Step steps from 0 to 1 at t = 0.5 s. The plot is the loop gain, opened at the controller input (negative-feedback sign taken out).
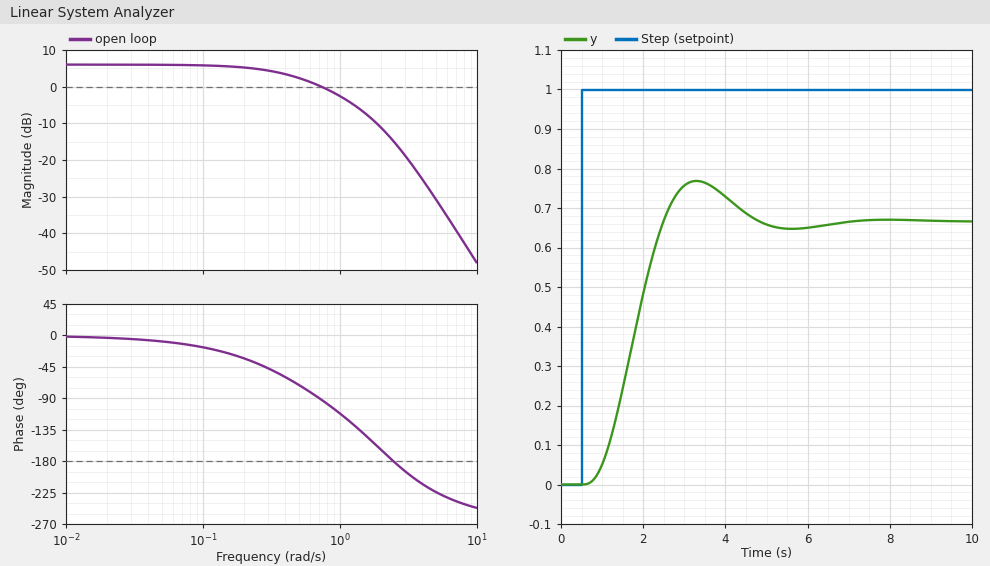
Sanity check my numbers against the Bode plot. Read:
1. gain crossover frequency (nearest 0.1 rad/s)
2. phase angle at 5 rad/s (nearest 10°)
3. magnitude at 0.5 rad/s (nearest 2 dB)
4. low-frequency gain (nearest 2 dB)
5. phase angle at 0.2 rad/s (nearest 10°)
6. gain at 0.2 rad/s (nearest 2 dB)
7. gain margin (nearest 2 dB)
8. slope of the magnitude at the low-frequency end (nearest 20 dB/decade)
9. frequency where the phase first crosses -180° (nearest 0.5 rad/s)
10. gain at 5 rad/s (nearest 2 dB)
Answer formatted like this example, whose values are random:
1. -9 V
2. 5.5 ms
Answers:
1. 0.7 rad/s
2. -220°
3. 2 dB
4. 6 dB
5. -30°
6. 6 dB
7. 14 dB
8. 0 dB/decade
9. 2.5 rad/s
10. -30 dB
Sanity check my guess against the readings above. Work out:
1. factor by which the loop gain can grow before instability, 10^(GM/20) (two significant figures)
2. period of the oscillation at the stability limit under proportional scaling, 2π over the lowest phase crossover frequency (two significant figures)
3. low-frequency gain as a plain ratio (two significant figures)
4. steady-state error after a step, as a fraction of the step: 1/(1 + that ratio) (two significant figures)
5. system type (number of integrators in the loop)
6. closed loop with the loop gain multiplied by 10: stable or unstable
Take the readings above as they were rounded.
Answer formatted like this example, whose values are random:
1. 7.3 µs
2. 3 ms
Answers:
1. 5.0
2. 2.5 s
3. 2.0
4. 0.33
5. 0
6. unstable
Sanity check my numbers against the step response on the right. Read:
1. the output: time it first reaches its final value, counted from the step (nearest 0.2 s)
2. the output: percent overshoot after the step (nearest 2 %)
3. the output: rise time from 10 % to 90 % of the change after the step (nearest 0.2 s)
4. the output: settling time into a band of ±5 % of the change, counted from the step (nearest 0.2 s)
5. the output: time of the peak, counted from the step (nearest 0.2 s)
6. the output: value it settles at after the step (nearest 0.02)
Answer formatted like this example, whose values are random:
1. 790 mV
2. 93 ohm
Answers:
1. 2.0 s
2. 16 %
3. 1.2 s
4. 3.8 s
5. 2.8 s
6. 0.66
